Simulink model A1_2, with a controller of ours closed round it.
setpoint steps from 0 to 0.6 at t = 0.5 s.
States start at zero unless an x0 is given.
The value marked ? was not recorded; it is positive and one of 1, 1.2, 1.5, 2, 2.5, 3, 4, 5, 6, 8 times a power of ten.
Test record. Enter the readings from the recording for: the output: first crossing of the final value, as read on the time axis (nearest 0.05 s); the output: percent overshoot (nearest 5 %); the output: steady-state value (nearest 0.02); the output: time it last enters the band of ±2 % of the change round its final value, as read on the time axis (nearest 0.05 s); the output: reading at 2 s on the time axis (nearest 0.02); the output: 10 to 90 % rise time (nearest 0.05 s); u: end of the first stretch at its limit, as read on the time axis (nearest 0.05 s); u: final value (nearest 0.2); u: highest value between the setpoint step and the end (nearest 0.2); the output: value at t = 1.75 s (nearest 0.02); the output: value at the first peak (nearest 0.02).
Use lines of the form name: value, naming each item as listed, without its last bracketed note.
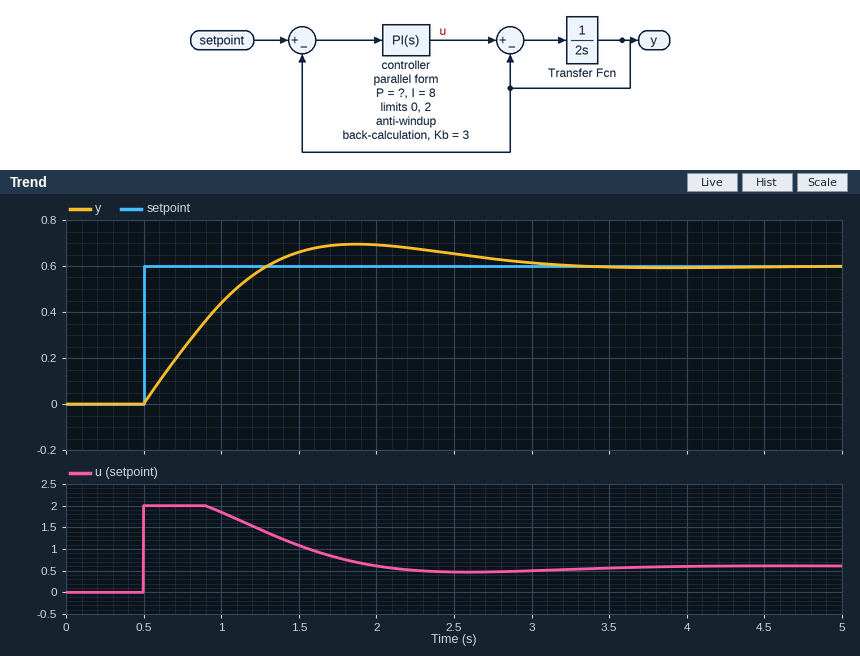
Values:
the output: first crossing of the final value, as read on the time axis: 1.30 s
the output: percent overshoot: 15 %
the output: steady-state value: 0.60
the output: time it last enters the band of ±2 % of the change round its final value, as read on the time axis: 3.05 s
the output: reading at 2 s on the time axis: 0.70
the output: 10 to 90 % rise time: 0.60 s
u: end of the first stretch at its limit, as read on the time axis: 0.90 s
u: final value: 0.6
u: highest value between the setpoint step and the end: 2.0
the output: value at t = 1.75 s: 0.70
the output: value at the first peak: 0.70
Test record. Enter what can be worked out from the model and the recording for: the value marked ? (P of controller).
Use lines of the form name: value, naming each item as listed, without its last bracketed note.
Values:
the value marked ?: 4
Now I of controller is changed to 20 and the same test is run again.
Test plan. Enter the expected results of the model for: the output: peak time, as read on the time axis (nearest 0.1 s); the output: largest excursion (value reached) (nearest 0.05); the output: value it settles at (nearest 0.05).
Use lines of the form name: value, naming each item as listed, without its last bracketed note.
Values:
the output: peak time, as read on the time axis: 1.6 s
the output: largest excursion (value reached): 0.75
the output: value it settles at: 0.60
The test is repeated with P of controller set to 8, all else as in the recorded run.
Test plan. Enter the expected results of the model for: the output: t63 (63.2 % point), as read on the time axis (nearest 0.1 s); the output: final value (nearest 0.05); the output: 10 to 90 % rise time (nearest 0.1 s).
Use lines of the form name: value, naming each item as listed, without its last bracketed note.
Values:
the output: t63 (63.2 % point), as read on the time axis: 0.9 s
the output: final value: 0.60
the output: 10 to 90 % rise time: 0.8 s
